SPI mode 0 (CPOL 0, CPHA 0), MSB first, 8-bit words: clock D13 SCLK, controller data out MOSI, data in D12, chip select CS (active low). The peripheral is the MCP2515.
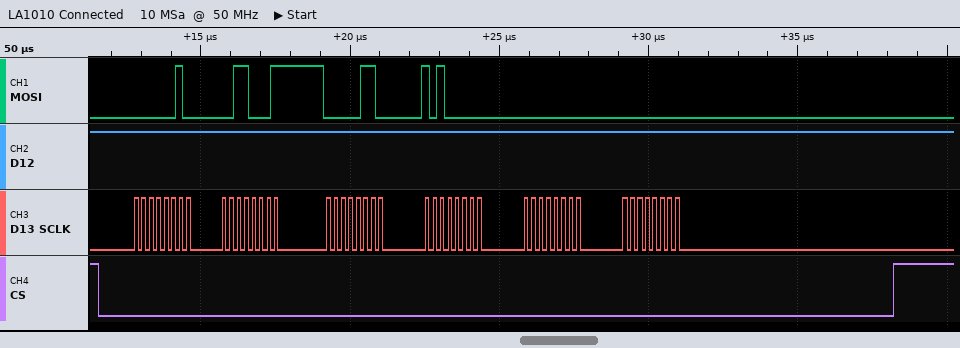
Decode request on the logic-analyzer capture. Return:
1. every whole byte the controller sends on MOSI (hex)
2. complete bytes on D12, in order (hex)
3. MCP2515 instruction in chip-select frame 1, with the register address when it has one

02 31 06 A0 00 00
FF FF FF FF FF FF
WRITE 0x31
